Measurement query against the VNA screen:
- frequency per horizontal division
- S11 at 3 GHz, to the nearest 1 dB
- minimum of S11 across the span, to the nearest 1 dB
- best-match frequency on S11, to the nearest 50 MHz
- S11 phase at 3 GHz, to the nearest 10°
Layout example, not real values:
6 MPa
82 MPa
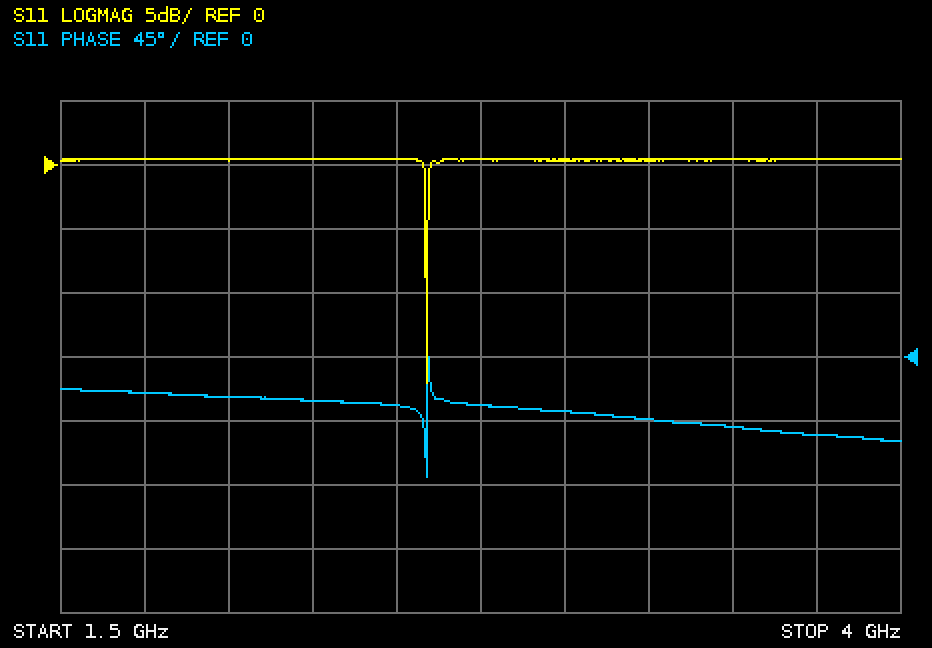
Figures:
250 MHz
0 dB
-17 dB
2.60 GHz
-40°
